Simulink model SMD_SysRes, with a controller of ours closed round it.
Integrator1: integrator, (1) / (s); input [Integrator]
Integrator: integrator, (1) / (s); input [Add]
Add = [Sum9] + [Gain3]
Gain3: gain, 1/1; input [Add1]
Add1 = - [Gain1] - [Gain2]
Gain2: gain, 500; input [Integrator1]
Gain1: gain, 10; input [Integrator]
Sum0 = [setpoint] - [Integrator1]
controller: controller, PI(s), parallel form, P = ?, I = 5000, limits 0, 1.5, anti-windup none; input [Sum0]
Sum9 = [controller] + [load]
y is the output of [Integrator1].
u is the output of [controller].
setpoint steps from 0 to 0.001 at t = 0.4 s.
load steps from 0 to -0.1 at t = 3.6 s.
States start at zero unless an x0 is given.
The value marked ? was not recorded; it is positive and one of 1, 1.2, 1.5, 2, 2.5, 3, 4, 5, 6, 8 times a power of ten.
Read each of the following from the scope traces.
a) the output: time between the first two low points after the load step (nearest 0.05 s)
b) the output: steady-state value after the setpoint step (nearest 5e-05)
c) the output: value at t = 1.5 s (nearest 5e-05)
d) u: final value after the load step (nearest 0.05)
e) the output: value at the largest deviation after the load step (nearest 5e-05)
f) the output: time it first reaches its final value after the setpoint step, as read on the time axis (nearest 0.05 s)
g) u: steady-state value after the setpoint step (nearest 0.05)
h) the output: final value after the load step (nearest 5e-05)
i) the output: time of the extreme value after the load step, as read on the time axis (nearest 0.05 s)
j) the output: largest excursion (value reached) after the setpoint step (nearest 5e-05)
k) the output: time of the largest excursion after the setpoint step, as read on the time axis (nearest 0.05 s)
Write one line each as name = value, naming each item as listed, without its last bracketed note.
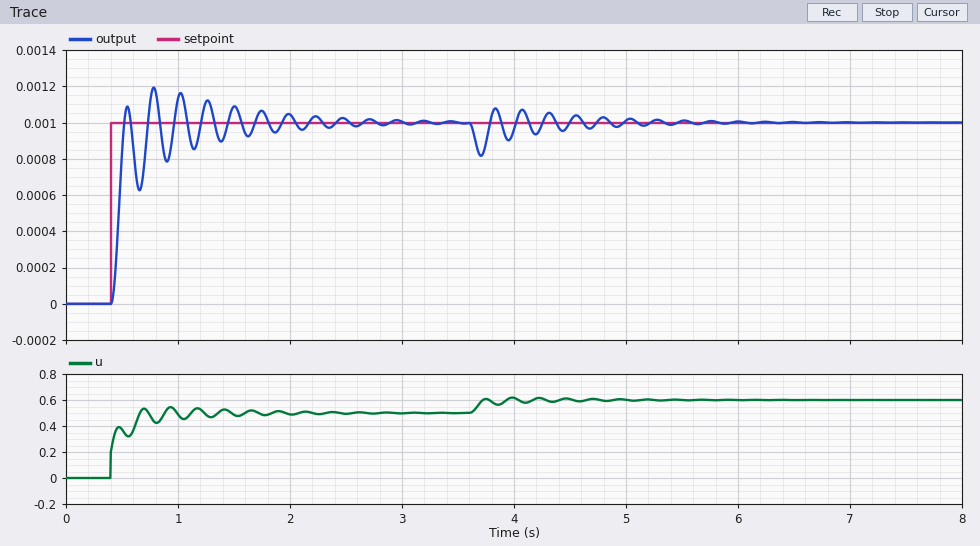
the output: time between the first two low points after the load step = 0.25 s
the output: steady-state value after the setpoint step = 0.00100
the output: value at t = 1.5 s = 0.00110
u: final value after the load step = 0.60
the output: value at the largest deviation after the load step = 0.00080
the output: time it first reaches its final value after the setpoint step, as read on the time axis = 0.50 s
u: steady-state value after the setpoint step = 0.50
the output: final value after the load step = 0.00100
the output: time of the extreme value after the load step, as read on the time axis = 3.70 s
the output: largest excursion (value reached) after the setpoint step = 0.00120
the output: time of the largest excursion after the setpoint step, as read on the time axis = 0.80 s
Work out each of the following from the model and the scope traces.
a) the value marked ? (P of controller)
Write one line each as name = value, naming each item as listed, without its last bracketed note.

the value marked ? = 200
